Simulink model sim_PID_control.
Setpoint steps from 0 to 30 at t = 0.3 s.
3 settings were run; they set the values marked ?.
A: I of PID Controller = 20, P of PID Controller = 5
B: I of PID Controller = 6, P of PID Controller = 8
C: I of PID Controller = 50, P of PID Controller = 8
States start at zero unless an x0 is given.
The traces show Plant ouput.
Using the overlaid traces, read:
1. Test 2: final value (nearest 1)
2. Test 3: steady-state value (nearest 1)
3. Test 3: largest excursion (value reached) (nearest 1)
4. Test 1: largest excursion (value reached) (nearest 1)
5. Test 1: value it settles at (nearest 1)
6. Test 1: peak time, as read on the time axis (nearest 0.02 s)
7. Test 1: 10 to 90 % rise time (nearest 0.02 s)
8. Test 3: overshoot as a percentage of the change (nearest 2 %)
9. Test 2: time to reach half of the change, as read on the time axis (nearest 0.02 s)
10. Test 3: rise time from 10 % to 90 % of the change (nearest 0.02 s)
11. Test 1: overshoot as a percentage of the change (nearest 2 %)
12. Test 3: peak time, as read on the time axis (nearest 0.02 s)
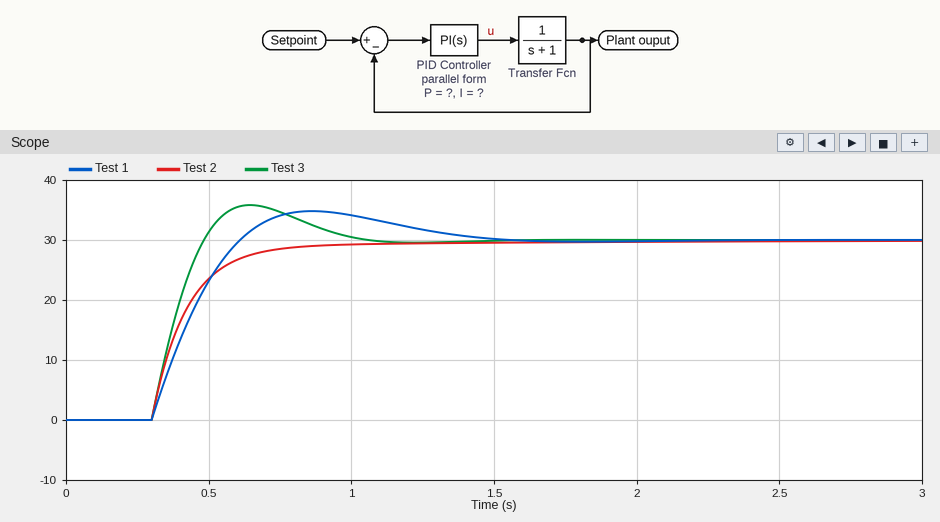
30
30
36
35
30
0.86 s
0.24 s
20 %
0.38 s
0.14 s
16 %
0.64 s
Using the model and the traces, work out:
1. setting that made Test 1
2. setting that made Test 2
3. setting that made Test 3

A
B
C
